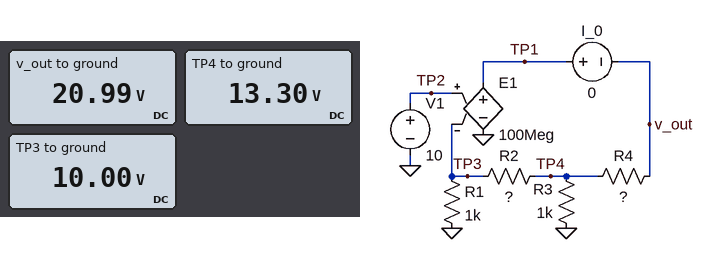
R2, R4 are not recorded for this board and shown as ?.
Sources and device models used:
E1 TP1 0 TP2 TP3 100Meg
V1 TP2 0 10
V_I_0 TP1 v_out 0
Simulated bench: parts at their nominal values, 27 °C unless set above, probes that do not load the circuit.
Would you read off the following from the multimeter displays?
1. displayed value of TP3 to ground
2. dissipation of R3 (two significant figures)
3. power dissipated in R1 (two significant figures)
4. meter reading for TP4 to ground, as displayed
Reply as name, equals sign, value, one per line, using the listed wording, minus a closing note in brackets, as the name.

displayed value of TP3 to ground = 10.00 V
dissipation of R3 = 180 mW
power dissipated in R1 = 100 mW
meter reading for TP4 to ground, as displayed = 13.30 V
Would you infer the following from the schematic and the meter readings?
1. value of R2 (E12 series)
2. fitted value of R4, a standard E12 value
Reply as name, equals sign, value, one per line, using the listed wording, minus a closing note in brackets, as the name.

value of R2 = 330 Ω
fitted value of R4, a standard E12 value = 330 Ω
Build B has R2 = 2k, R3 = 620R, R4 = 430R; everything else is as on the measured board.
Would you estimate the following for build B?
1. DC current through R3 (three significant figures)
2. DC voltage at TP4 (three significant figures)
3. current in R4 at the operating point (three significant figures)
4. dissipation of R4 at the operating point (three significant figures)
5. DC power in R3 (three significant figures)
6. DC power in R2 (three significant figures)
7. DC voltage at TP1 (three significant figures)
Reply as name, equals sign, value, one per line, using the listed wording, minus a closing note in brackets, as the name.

DC current through R3 = 48.4 mA
DC voltage at TP4 = 30.0 V
current in R4 at the operating point = 58.4 mA
dissipation of R4 at the operating point = 1.47 W
DC power in R3 = 1.45 W
DC power in R2 = 200 mW
DC voltage at TP1 = 55.1 V
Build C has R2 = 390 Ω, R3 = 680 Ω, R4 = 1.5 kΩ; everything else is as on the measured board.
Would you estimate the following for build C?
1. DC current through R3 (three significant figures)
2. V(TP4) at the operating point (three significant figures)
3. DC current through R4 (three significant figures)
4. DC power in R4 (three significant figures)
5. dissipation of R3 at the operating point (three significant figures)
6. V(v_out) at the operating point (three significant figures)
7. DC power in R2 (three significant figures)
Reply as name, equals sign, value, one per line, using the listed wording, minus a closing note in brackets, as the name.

DC current through R3 = 20.4 mA
V(TP4) at the operating point = 13.9 V
DC current through R4 = 30.4 mA
DC power in R4 = 1.39 W
dissipation of R3 at the operating point = 284 mW
V(v_out) at the operating point = 59.6 V
DC power in R2 = 39.0 mW
